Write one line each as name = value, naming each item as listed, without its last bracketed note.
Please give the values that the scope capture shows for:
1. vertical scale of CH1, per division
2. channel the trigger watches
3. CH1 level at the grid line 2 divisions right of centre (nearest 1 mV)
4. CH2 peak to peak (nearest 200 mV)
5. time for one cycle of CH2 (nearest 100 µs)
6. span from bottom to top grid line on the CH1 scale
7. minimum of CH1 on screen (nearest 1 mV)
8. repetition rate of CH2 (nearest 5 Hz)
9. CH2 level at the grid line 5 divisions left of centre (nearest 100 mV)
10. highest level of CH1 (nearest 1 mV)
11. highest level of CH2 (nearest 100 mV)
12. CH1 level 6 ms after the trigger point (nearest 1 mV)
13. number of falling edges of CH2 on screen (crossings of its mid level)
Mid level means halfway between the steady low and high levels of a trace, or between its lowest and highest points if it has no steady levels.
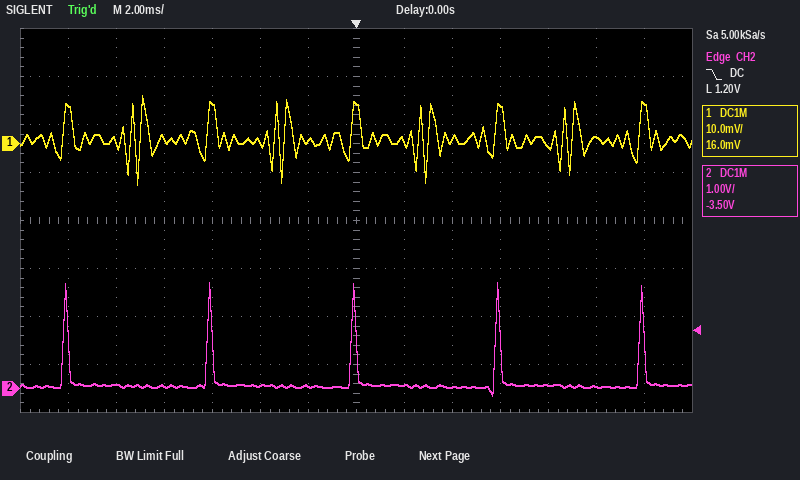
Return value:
vertical scale of CH1, per division = 10 mV
channel the trigger watches = CH2
CH1 level at the grid line 2 divisions right of centre = 1 mV
CH2 peak to peak = 2.4 V
time for one cycle of CH2 = 6.0 ms
span from bottom to top grid line on the CH1 scale = 80 mV
minimum of CH1 on screen = -8 mV
repetition rate of CH2 = 165 Hz
CH2 level at the grid line 5 divisions left of centre = 100 mV
highest level of CH1 = 10 mV
highest level of CH2 = 2.2 V
CH1 level 6 ms after the trigger point = 8 mV
number of falling edges of CH2 on screen = 5
